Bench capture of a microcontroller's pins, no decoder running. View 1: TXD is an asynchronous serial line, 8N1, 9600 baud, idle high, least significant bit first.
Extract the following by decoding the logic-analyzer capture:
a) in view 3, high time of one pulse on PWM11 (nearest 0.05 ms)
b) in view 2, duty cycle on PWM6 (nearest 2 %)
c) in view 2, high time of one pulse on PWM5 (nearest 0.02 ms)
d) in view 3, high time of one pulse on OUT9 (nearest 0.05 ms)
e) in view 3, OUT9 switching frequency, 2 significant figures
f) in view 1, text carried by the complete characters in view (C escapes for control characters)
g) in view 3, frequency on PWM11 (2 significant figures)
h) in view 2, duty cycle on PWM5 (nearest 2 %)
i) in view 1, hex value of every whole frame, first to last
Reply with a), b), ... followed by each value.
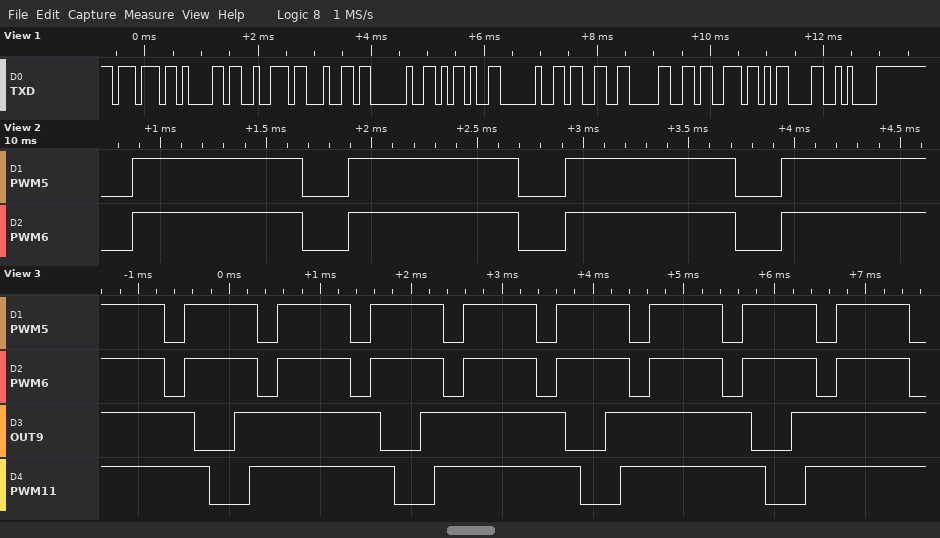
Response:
a) 1.60 ms
b) 78 %
c) 0.80 ms
d) 1.60 ms
e) 490 Hz
f) "ward - 30s\r\n"
g) 490 Hz
h) 78 %
i) 0x77 0x61 0x72 0x64 0x20 0x2D 0x20 0x33 0x30 0x73 0x0D 0x0A
